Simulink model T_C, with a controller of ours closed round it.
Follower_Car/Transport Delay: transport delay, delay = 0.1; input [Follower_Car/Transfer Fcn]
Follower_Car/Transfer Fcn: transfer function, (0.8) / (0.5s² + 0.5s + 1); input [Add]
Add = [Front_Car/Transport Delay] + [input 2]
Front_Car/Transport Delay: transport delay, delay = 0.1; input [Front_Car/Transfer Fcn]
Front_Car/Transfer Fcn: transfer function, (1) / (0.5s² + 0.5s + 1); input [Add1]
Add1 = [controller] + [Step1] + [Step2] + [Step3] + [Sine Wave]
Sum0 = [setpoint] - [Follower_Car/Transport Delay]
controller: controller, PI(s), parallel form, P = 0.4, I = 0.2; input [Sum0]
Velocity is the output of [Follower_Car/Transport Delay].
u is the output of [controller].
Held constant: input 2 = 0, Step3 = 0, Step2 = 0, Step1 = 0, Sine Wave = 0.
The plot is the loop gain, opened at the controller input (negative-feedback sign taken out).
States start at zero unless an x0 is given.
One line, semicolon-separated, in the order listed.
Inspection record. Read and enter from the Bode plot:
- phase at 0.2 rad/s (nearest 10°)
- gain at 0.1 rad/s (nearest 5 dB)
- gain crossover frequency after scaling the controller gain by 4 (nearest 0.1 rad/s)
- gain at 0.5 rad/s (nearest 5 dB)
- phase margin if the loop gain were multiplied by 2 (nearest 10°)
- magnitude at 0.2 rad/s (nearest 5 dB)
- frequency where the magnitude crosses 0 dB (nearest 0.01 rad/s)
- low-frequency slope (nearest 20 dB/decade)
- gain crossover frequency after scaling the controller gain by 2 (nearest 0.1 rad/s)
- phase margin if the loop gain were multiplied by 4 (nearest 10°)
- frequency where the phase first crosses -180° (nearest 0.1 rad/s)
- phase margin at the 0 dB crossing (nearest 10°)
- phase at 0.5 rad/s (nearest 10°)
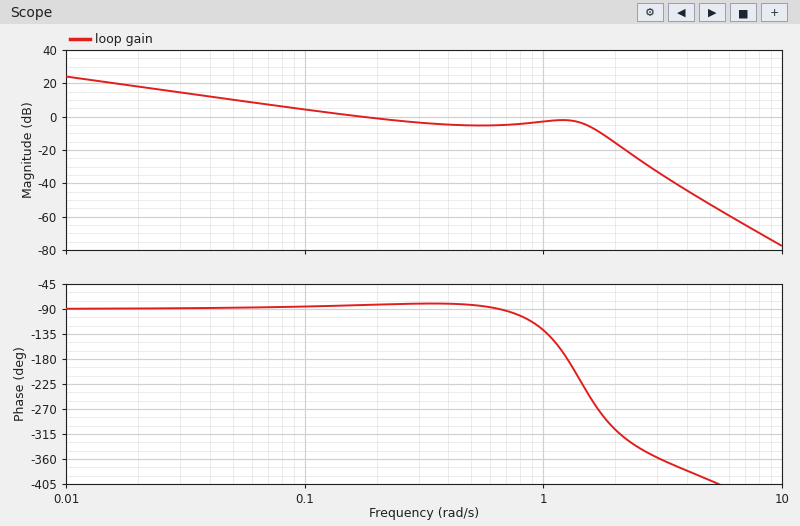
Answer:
-80°; 5 dB; 1.8 rad/s; -5 dB; -70°; 0 dB; 0.17 rad/s; -20 dB/decade; 1.6 rad/s; -110°; 1.3 rad/s; 100°; -80°
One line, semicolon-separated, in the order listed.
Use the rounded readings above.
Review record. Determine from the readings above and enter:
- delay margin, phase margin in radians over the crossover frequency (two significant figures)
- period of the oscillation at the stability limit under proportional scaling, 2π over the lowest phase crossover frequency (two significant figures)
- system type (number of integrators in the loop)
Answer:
10 s; 4.8 s; 1
